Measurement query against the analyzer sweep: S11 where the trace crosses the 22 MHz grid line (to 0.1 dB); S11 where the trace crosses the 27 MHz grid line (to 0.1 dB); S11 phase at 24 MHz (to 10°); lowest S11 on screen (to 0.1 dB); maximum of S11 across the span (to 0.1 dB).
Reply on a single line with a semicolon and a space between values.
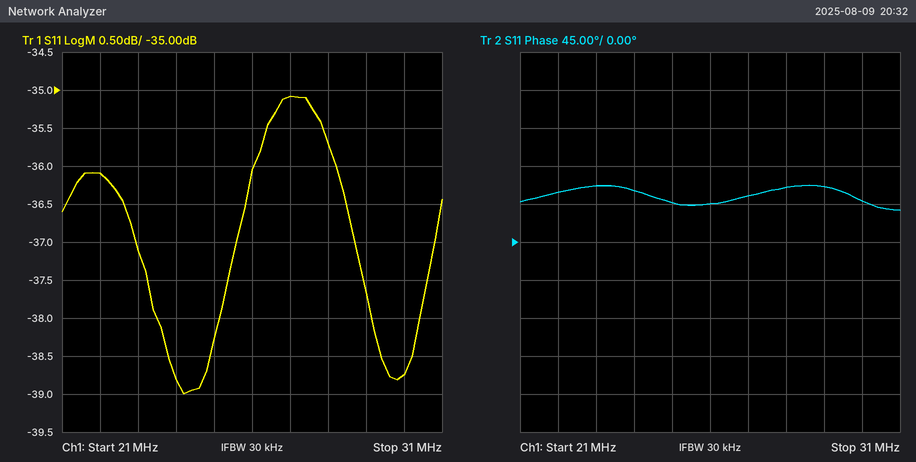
-36.1 dB; -35.1 dB; 60°; -39.0 dB; -35.1 dB
